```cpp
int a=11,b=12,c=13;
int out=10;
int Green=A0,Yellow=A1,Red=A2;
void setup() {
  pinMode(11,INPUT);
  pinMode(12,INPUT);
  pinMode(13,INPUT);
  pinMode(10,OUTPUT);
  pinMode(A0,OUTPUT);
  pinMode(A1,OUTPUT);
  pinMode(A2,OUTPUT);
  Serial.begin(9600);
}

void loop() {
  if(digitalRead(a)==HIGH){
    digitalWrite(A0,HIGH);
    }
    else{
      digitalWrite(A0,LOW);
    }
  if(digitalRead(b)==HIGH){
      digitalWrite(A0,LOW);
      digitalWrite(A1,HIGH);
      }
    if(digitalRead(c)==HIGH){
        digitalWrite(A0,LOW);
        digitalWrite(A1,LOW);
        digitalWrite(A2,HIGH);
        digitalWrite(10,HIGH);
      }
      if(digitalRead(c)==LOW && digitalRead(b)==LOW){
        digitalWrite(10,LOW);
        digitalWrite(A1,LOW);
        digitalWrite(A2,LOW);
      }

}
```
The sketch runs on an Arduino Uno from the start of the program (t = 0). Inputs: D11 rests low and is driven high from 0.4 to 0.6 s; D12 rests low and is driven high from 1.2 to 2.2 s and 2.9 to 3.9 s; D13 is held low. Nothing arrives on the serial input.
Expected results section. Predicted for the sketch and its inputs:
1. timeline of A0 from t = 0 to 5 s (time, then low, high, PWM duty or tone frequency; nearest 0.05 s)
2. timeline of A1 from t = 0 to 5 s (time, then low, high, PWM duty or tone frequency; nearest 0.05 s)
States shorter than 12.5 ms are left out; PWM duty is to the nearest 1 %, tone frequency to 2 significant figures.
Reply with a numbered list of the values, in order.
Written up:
1. 0 s low; 0.4 s high; 0.6 s low
2. 0 s low; 1.2 s high; 2.2 s low; 2.9 s high; 3.9 s low
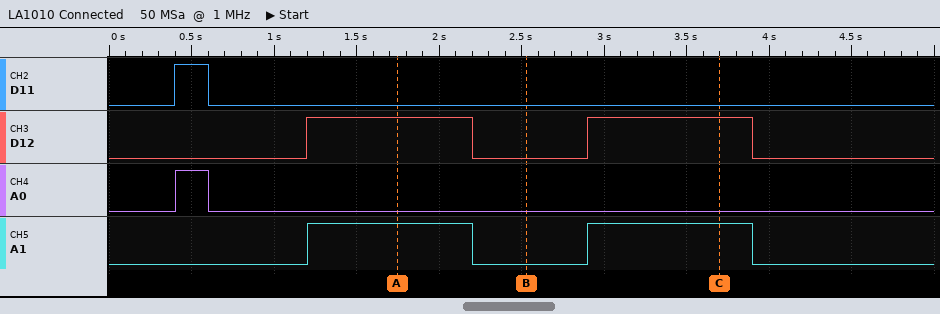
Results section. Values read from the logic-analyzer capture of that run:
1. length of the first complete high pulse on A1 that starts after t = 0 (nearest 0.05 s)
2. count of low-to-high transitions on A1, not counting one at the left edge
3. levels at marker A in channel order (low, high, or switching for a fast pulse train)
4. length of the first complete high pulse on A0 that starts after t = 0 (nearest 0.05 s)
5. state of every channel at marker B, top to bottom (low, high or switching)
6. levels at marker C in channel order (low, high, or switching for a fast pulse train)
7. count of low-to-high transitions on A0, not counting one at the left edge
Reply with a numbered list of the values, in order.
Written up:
1. 1.00 s
2. 2
3. D11 low, D12 high, A0 low, A1 high
4. 0.20 s
5. D11 low, D12 low, A0 low, A1 low
6. D11 low, D12 high, A0 low, A1 high
7. 1
